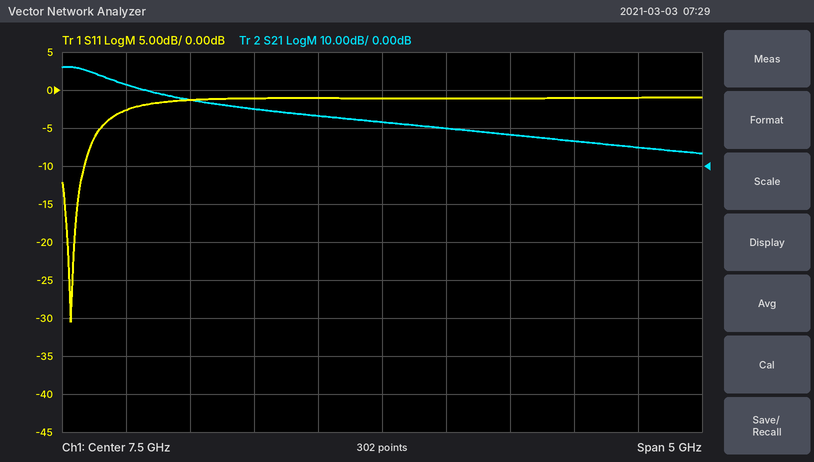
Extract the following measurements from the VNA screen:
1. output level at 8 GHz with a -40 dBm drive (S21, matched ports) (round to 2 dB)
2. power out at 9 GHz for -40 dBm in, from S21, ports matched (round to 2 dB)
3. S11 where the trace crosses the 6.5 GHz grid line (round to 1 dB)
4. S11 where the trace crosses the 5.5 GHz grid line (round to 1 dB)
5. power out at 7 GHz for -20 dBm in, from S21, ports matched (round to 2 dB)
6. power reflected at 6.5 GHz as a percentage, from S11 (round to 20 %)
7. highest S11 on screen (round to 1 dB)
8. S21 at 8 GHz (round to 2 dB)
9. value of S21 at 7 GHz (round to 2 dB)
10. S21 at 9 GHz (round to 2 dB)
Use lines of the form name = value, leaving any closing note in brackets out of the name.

output level at 8 GHz with a -40 dBm drive (S21, matched ports) = -30 dBm
power out at 9 GHz for -40 dBm in, from S21, ports matched = -34 dBm
S11 where the trace crosses the 6.5 GHz grid line = -1 dB
S11 where the trace crosses the 5.5 GHz grid line = -3 dB
power out at 7 GHz for -20 dBm in, from S21, ports matched = -6 dBm
power reflected at 6.5 GHz as a percentage, from S11 = 80 %
highest S11 on screen = -1 dB
S21 at 8 GHz = 10 dB
value of S21 at 7 GHz = 14 dB
S21 at 9 GHz = 6 dB
